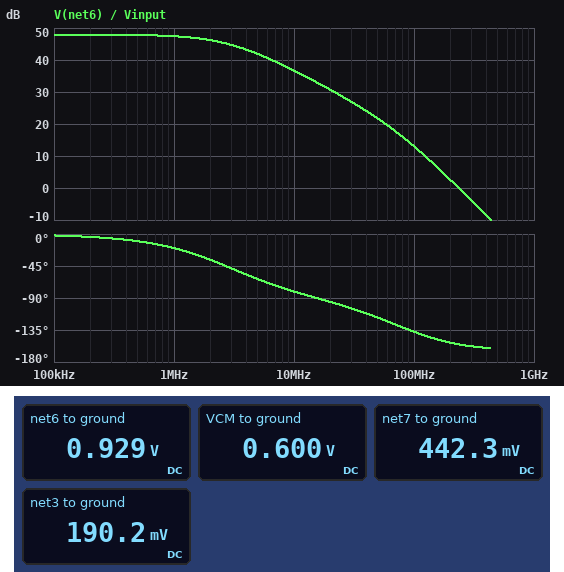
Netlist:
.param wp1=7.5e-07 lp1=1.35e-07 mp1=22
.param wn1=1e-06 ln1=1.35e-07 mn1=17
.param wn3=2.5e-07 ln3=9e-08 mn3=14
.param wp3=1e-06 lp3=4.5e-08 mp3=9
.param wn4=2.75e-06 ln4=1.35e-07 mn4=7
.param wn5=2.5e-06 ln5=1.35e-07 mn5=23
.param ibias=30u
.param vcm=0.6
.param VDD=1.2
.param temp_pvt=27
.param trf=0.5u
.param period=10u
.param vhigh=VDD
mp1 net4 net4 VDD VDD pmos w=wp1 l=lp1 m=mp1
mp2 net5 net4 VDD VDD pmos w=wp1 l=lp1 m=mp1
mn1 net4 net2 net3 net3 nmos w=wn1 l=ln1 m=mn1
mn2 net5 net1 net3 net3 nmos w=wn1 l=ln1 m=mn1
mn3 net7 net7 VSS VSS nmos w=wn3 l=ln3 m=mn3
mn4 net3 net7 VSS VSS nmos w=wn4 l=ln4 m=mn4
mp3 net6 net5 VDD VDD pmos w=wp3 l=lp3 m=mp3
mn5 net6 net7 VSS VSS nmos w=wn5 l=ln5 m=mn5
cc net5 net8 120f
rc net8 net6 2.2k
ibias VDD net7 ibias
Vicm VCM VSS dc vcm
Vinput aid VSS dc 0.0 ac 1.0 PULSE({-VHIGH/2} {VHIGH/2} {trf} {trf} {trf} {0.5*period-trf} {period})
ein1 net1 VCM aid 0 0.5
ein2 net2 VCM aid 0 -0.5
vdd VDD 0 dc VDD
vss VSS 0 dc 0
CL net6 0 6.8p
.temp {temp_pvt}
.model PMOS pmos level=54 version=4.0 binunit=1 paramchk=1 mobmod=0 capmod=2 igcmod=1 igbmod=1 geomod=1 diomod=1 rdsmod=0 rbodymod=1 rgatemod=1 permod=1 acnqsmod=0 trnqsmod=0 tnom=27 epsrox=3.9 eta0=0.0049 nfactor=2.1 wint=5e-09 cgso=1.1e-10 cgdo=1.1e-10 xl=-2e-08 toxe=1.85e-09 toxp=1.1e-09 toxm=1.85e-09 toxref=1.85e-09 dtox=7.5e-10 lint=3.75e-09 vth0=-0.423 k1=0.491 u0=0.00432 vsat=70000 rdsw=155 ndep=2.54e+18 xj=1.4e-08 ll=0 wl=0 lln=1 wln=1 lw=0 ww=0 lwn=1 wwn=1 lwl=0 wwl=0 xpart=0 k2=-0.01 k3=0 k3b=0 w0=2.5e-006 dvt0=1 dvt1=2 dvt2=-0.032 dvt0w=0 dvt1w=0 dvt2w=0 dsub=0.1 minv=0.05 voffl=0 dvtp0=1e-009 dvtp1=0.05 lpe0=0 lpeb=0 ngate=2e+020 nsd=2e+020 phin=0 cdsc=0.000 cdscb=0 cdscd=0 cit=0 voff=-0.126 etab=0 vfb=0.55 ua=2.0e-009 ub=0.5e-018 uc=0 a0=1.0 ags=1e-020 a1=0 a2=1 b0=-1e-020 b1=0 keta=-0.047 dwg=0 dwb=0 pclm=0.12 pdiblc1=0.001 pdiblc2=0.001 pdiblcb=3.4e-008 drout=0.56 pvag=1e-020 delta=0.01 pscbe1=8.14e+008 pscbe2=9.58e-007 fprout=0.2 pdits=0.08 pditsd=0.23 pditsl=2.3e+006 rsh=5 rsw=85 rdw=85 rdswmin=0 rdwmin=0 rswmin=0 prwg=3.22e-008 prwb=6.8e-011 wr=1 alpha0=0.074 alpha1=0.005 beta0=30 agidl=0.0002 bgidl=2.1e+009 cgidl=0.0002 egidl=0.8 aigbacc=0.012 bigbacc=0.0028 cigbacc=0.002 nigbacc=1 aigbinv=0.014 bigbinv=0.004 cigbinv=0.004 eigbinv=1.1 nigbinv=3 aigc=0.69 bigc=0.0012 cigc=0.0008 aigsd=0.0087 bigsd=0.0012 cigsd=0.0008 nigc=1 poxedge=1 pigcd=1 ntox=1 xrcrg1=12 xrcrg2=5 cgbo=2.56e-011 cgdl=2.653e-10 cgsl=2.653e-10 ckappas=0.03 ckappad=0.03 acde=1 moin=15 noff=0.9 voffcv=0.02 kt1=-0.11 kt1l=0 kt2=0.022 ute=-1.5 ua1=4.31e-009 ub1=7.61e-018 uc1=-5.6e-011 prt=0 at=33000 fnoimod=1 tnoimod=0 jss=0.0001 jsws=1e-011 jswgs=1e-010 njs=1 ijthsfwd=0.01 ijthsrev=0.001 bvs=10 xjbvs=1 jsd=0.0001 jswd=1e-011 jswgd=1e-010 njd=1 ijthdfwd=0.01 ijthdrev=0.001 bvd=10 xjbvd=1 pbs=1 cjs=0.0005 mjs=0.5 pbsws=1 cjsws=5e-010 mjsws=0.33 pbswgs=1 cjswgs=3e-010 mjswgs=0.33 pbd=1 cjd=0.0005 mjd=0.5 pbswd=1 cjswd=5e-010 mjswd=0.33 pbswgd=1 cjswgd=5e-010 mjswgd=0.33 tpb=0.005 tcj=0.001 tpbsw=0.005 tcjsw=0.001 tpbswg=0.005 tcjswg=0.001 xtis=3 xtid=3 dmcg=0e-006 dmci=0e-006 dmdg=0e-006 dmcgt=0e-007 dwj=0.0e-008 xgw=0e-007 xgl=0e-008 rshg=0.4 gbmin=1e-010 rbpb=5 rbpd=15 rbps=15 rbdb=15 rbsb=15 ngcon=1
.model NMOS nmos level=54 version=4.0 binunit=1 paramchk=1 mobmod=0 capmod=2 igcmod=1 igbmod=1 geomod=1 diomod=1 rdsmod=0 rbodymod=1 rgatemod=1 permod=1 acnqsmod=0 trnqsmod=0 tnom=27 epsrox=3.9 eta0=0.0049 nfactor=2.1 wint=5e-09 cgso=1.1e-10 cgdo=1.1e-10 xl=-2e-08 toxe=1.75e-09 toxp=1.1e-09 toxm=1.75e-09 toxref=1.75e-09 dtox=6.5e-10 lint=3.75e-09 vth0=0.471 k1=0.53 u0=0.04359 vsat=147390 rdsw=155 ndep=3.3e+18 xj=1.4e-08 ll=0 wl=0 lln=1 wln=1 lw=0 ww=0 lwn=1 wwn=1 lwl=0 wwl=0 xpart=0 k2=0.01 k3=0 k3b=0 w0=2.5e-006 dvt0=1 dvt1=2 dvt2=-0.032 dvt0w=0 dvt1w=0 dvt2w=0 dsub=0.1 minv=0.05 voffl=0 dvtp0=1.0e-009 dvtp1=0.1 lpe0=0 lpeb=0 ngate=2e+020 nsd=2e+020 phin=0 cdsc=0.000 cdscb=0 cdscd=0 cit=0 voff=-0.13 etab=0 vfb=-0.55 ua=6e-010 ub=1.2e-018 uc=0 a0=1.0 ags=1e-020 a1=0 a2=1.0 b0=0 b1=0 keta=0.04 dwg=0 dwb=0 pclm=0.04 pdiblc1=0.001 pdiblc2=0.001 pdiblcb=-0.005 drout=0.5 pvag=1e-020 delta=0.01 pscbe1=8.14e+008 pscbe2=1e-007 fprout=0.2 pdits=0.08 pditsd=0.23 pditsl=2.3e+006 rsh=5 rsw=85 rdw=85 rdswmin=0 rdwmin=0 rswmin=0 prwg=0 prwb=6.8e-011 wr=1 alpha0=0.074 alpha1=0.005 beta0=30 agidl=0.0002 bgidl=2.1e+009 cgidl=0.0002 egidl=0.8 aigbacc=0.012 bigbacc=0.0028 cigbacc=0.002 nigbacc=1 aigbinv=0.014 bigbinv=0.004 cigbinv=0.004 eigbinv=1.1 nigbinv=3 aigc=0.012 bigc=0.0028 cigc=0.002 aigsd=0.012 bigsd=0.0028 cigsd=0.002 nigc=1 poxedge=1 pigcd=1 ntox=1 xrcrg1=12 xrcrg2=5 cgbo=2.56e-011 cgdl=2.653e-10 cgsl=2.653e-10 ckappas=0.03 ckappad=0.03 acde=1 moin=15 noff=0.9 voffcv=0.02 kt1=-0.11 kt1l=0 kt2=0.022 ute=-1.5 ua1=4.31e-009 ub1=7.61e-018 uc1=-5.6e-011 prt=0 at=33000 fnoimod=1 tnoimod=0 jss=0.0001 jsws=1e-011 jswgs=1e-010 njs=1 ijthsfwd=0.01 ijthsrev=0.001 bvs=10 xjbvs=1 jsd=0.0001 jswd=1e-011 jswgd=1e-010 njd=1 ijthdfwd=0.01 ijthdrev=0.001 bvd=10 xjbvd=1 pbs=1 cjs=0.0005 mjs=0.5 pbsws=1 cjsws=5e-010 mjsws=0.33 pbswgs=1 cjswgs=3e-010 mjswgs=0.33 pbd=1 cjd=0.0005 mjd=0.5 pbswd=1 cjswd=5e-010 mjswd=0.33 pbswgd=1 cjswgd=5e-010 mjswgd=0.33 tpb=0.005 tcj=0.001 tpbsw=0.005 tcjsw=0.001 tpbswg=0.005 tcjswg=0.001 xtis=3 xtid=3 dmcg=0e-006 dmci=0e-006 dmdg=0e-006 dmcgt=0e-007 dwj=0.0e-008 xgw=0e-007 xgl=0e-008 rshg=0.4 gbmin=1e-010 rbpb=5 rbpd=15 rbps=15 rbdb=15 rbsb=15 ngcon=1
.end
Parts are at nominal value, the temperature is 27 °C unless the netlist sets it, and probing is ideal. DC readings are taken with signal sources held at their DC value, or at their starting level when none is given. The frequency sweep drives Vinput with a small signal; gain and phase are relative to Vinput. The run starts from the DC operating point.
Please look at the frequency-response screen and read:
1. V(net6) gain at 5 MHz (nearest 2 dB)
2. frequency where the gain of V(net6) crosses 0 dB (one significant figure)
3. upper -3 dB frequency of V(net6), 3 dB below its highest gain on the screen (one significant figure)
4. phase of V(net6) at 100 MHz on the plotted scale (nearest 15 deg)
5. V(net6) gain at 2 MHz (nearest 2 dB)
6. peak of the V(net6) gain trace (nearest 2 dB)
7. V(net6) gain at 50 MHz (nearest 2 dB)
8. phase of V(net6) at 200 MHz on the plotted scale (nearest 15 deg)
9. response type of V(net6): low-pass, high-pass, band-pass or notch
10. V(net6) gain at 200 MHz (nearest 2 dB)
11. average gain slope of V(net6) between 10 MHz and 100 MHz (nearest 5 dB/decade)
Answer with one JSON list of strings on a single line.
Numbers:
["42 dB", "200 MHz", "3 MHz", "-135 deg", "46 dB", "48 dB", "22 dB", "-150 deg", "low-pass", "2 dB", "-25 dB/decade"]
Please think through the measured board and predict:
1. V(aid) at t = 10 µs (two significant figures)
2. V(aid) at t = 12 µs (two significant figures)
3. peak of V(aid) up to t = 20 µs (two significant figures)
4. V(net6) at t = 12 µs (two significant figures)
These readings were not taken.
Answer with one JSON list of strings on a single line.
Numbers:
["-600 mV", "600 mV", "600 mV", "1.2 V"]
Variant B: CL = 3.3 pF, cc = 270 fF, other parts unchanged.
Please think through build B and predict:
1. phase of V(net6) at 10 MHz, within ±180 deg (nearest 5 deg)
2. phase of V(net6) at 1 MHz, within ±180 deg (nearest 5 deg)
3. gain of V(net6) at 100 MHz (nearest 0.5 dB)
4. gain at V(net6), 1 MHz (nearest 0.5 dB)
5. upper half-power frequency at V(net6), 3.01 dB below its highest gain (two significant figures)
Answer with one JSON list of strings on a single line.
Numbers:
["-85 deg", "-35 deg", "10.5 dB", "46.5 dB", "1.5 MHz"]
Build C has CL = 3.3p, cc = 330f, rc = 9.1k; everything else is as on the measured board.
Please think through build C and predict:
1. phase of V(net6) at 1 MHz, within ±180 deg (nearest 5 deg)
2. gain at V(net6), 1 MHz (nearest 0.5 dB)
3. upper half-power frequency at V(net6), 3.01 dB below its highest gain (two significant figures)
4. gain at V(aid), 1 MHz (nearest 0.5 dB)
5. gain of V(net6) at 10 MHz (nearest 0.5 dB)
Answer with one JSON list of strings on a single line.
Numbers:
["-40 deg", "45.5 dB", "1.2 MHz", "0 dB", "29.5 dB"]
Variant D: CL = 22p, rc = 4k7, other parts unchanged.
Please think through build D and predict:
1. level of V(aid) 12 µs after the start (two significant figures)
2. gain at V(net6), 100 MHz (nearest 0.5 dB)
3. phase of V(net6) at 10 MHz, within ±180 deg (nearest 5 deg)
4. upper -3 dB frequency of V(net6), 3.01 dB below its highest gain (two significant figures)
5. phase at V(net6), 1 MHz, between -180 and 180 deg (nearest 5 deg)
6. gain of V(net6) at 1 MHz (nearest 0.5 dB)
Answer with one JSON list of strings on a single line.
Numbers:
["600 mV", "5.0 dB", "-95 deg", "2.2 MHz", "-25 deg", "47.0 dB"]
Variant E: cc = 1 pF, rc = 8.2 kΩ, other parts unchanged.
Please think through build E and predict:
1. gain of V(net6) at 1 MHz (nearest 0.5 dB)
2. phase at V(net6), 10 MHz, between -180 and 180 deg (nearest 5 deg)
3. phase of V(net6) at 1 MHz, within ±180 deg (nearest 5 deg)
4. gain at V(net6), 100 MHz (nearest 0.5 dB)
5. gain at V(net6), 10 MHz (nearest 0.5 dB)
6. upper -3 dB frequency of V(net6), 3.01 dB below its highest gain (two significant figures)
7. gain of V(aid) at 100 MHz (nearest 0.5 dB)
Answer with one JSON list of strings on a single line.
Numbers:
["39.5 dB", "-70 deg", "-65 deg", "10.5 dB", "21.0 dB", "410 kHz", "0 dB"]
